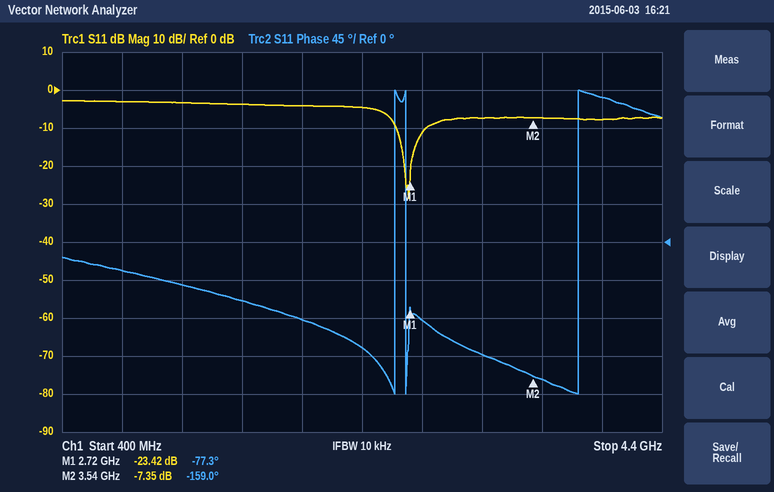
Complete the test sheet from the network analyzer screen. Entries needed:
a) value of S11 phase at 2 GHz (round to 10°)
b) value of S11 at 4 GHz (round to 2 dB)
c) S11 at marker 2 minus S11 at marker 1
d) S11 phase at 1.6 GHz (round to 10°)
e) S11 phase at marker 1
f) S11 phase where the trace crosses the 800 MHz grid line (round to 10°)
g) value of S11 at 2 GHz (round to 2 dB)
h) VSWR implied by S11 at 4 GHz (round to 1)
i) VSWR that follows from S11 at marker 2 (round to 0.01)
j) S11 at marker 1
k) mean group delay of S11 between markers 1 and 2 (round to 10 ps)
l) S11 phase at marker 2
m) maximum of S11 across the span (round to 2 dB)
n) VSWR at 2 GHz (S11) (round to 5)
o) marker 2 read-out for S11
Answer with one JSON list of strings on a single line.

["-90°", "-8 dB", "16.07 dB", "-70°", "-77.3°", "-30°", "-4 dB", "2", "2.50", "-23.42 dB", "280 ps", "-159.0°", "-2 dB", "5", "-7.35 dB"]
